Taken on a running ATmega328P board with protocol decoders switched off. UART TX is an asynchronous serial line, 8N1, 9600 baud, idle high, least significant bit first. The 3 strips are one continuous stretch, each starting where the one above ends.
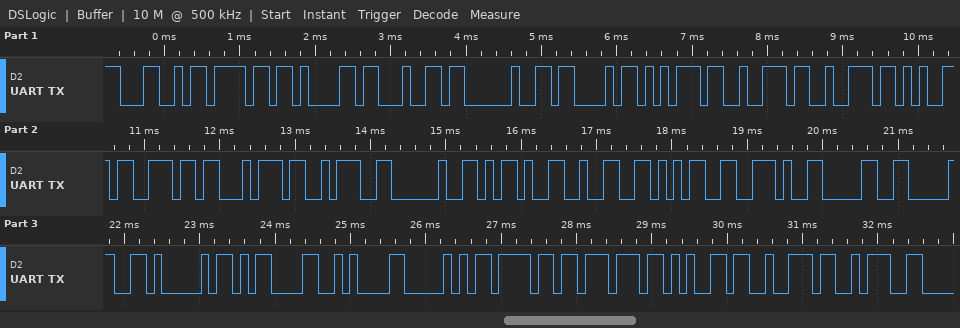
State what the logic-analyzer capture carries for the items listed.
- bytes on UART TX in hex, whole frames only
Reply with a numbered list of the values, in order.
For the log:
1. 4C 6F 61 64 20 43 75 72 72 65 6E 74 3A 20 2D 32 35 2E 30 30 41 0D 0A 50 6F 77 65 72 3A
